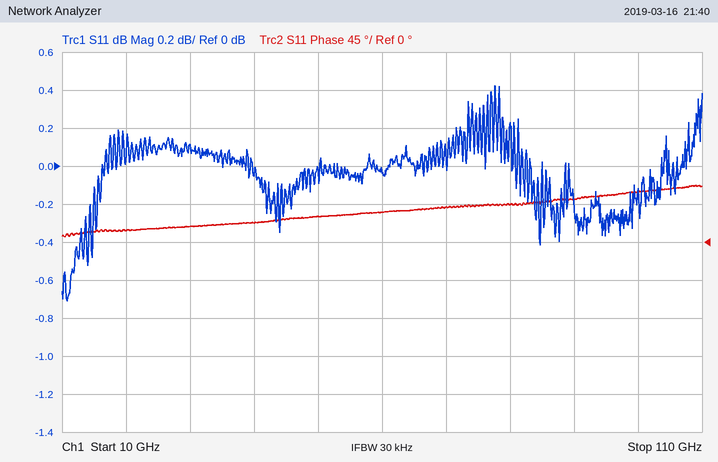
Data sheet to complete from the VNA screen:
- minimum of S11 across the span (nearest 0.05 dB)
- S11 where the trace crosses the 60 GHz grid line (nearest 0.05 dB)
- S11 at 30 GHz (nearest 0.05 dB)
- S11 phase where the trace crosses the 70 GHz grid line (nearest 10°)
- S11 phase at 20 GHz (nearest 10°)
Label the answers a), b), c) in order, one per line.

a) -0.70 dB
b) -0.05 dB
c) 0.10 dB
d) 40°
e) 10°
